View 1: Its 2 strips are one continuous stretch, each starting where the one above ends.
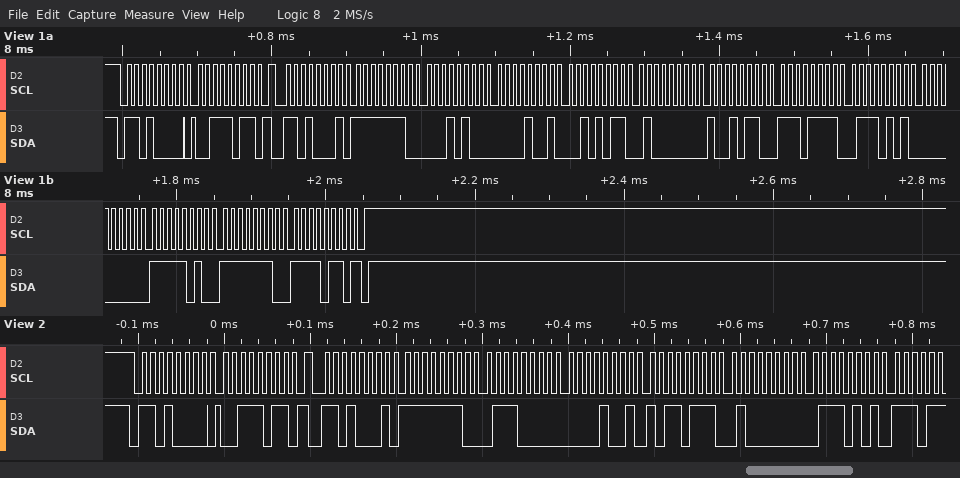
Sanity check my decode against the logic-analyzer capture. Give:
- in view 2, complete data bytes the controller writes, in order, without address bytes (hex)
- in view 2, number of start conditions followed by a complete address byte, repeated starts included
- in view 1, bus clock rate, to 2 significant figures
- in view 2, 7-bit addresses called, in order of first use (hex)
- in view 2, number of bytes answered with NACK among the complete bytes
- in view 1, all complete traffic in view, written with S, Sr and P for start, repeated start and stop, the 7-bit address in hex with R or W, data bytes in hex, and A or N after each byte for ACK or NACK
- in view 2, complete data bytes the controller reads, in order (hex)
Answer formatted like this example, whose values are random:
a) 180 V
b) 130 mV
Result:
a) 3B
b) 2
c) 100 kHz
d) 0x68
e) 0
f) S 68W A 3B A Sr 68R A FE A 14 A 09 A 2B A 40 A 96 A EF A 75 A 00 A FA A FE A F6 N P
g) FE 70 09 B7 40 75
